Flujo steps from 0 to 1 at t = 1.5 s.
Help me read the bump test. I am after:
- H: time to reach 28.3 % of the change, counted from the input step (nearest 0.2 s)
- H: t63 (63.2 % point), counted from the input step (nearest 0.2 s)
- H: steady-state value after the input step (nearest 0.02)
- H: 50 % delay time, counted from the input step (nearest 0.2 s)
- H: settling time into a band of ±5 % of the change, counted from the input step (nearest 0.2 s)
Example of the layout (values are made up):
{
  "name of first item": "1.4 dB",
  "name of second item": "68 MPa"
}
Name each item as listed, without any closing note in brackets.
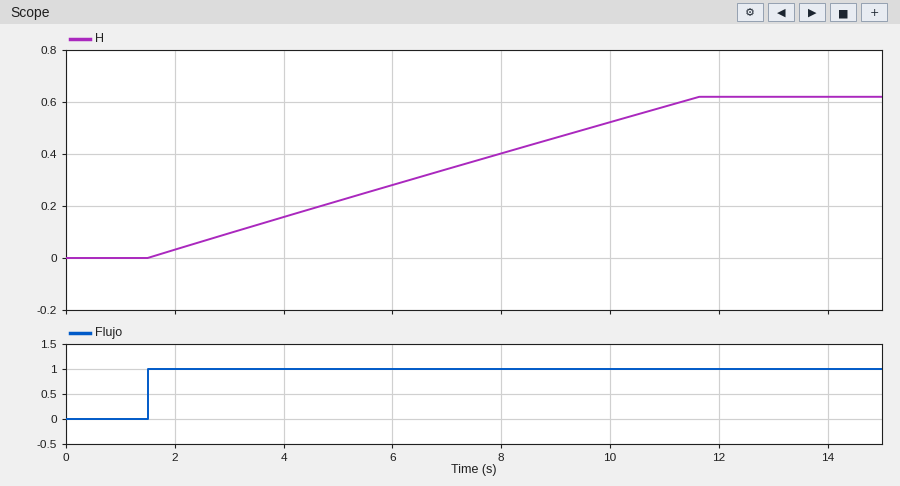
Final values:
{
  "H: time to reach 28.3 % of the change, counted from the input step": "2.8 s",
  "H: t63 (63.2 % point), counted from the input step": "6.4 s",
  "H: steady-state value after the input step": "0.62",
  "H: 50 % delay time, counted from the input step": "5.0 s",
  "H: settling time into a band of ±5 % of the change, counted from the input step": "9.6 s"
}
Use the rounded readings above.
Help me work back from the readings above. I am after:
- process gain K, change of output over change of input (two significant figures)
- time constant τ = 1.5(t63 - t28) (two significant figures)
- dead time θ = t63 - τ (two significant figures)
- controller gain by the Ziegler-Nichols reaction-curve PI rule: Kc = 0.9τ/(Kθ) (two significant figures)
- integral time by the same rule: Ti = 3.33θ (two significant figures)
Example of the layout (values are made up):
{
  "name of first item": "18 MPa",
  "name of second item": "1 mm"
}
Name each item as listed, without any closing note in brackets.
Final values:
{
  "process gain K, change of output over change of input": "0.62",
  "time constant τ = 1.5(t63 - t28)": "5.4 s",
  "dead time θ = t63 - τ": "1.0 s",
  "controller gain by the Ziegler-Nichols reaction-curve PI rule: Kc = 0.9τ/(Kθ)": "7.8",
  "integral time by the same rule: Ti = 3.33θ": "3.3 s"
}
